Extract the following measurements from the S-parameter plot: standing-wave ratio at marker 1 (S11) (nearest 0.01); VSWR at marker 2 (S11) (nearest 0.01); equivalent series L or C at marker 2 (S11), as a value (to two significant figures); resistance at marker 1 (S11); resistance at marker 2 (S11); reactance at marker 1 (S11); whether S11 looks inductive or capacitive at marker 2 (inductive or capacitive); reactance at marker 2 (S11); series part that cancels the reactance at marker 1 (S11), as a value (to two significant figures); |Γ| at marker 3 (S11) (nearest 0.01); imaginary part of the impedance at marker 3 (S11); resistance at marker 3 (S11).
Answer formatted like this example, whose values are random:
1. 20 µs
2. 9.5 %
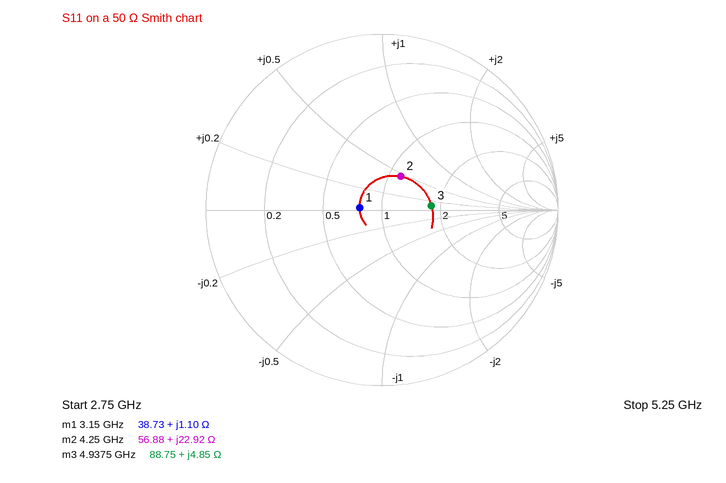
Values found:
1. 1.29
2. 1.56
3. 860 pH
4. 38.73 Ω
5. 56.88 Ω
6. +1.10 Ω
7. inductive
8. +22.92 Ω
9. 46 pF
10. 0.28
11. +4.85 Ω
12. 88.75 Ω
